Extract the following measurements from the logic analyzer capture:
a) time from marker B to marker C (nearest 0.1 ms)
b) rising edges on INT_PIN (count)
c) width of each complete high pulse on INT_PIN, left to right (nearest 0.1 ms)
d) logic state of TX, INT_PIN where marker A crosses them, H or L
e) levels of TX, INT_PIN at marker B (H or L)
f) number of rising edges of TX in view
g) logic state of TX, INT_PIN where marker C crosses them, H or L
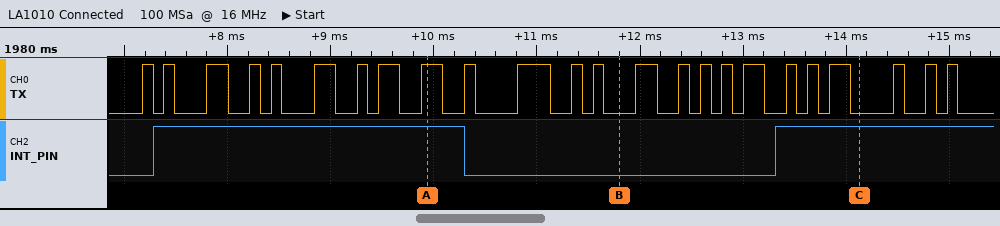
2.3 ms
2
3 ms
TX=H, INT_PIN=H
TX=L, INT_PIN=L
24
TX=L, INT_PIN=H
